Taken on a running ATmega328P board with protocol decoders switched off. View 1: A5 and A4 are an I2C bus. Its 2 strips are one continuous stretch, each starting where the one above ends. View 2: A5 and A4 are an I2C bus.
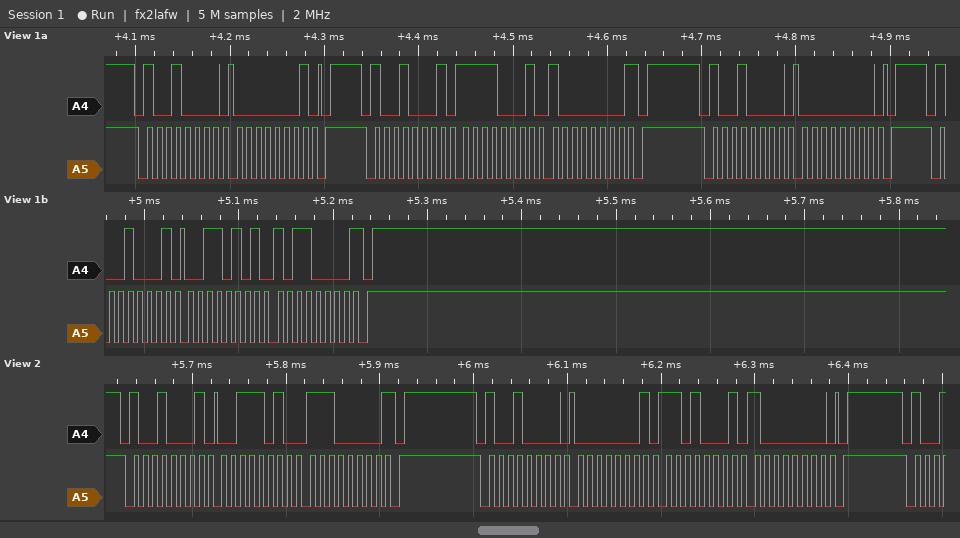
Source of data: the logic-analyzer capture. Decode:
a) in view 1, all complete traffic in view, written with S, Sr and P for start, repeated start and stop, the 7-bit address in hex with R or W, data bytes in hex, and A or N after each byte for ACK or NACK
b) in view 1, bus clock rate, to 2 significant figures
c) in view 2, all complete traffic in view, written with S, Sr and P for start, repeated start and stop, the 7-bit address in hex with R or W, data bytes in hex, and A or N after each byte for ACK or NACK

S 48W A 01 A P S 48R A F1 A 80 N P S 48W A 00 A P S 48R A 35 A B0 N P
100 kHz
S 48R A 3A A E0 N P S 48W A 01 A D1 A 80 A P
